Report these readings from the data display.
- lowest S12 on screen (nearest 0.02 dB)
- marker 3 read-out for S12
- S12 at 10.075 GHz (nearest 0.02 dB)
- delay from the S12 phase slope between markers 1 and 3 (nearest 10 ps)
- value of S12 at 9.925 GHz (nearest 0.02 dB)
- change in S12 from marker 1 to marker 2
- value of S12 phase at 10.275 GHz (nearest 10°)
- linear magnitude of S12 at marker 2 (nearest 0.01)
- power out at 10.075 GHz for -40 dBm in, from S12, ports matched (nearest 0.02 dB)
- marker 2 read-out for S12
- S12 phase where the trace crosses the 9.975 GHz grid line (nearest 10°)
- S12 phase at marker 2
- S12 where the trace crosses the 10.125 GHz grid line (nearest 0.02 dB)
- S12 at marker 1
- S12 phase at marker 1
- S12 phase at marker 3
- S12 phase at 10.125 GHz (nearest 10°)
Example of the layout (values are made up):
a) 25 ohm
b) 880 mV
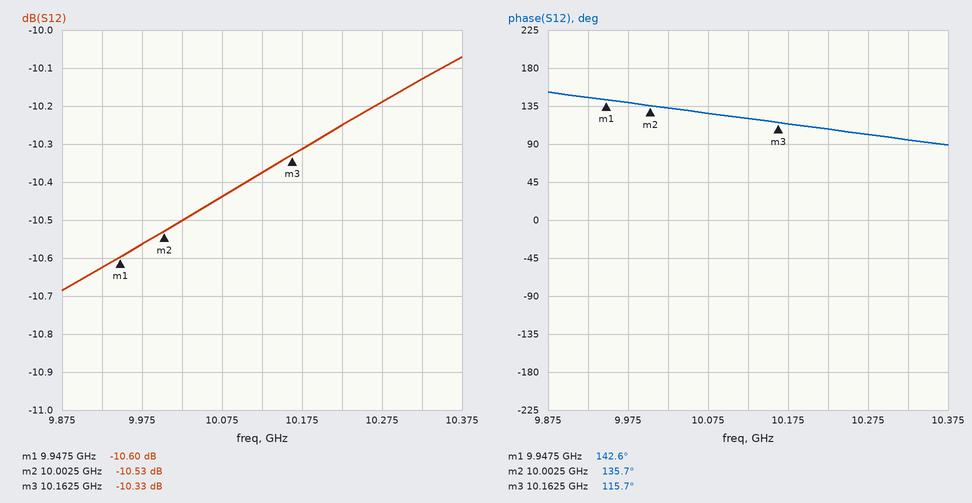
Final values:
a) -10.68 dB
b) -10.33 dB
c) -10.44 dB
d) 350 ps
e) -10.62 dB
f) 0.07 dB
g) 100°
h) 0.30
i) -50.44 dBm
j) -10.53 dB
k) 140°
l) 135.7°
m) -10.38 dB
n) -10.60 dB
o) 142.6°
p) 115.7°
q) 120°
